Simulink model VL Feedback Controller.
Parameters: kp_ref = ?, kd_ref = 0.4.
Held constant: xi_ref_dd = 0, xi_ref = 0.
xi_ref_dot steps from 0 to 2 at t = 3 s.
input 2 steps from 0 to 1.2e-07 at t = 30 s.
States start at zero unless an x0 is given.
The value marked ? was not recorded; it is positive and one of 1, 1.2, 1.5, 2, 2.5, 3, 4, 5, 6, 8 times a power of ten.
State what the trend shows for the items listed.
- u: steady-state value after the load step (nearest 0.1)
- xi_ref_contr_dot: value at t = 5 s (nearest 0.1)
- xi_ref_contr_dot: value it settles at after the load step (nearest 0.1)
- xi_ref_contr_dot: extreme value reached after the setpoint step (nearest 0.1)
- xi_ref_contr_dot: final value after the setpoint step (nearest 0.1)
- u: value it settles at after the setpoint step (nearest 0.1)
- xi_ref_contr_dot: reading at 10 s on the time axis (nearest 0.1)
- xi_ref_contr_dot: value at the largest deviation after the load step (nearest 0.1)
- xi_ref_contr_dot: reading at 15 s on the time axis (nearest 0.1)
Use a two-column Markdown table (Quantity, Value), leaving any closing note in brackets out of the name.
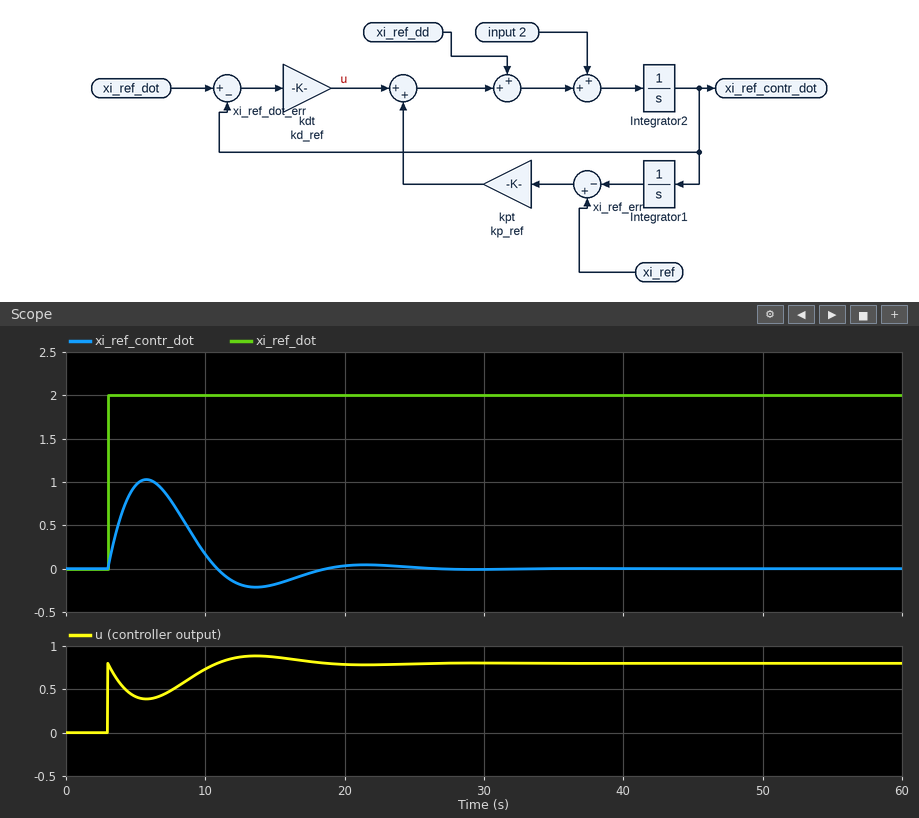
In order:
| Quantity | Value |
|---|---|
| u: steady-state value after the load step | 0.8 |
| xi_ref_contr_dot: value at t = 5 s | 1.0 |
| xi_ref_contr_dot: value it settles at after the load step | 0.0 |
| xi_ref_contr_dot: extreme value reached after the setpoint step | 1.0 |
| xi_ref_contr_dot: final value after the setpoint step | 0.0 |
| u: value it settles at after the setpoint step | 0.8 |
| xi_ref_contr_dot: reading at 10 s on the time axis | 0.2 |
| xi_ref_contr_dot: value at the largest deviation after the load step | 0.0 |
| xi_ref_contr_dot: reading at 15 s on the time axis | -0.2 |
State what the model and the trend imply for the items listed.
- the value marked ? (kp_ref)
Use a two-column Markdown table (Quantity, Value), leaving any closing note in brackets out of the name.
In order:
| Quantity | Value |
|---|---|
| the value marked ? | 0.2 |
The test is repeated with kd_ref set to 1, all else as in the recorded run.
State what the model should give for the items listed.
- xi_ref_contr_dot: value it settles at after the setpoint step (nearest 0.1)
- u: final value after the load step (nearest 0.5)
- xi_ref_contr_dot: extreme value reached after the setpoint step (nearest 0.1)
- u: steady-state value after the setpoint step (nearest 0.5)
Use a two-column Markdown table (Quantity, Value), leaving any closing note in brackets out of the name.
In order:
| Quantity | Value |
|---|---|
| xi_ref_contr_dot: value it settles at after the setpoint step | 0.0 |
| u: final value after the load step | 2.0 |
| xi_ref_contr_dot: extreme value reached after the setpoint step | 1.5 |
| u: steady-state value after the setpoint step | 2.0 |
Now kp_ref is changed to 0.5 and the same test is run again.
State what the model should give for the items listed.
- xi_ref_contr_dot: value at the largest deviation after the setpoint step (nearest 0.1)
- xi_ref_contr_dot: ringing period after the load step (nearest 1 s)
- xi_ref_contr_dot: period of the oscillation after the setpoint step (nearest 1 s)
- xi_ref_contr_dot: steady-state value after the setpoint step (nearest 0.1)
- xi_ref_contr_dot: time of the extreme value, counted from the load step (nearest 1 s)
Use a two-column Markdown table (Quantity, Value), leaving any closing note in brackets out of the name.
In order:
| Quantity | Value |
|---|---|
| xi_ref_contr_dot: value at the largest deviation after the setpoint step | 0.8 |
| xi_ref_contr_dot: ringing period after the load step | 9 s |
| xi_ref_contr_dot: period of the oscillation after the setpoint step | 9 s |
| xi_ref_contr_dot: steady-state value after the setpoint step | 0.0 |
| xi_ref_contr_dot: time of the extreme value, counted from the load step | 3 s |
